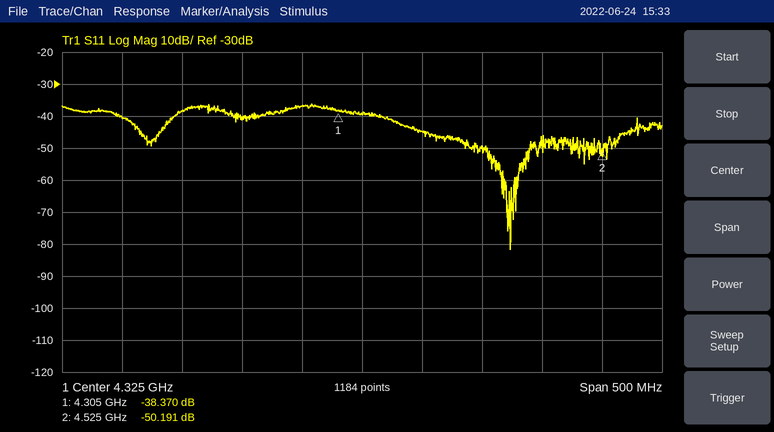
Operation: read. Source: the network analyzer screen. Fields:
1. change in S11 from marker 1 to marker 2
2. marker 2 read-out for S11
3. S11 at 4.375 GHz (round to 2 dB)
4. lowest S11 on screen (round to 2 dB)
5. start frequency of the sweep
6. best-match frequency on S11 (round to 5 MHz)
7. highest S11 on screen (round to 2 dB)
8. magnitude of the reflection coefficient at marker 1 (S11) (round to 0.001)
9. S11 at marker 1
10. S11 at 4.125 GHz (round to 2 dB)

-11.821 dB
-50.191 dB
-44 dB
-82 dB
4.075 GHz
4.450 GHz
-36 dB
0.012
-38.370 dB
-40 dB
